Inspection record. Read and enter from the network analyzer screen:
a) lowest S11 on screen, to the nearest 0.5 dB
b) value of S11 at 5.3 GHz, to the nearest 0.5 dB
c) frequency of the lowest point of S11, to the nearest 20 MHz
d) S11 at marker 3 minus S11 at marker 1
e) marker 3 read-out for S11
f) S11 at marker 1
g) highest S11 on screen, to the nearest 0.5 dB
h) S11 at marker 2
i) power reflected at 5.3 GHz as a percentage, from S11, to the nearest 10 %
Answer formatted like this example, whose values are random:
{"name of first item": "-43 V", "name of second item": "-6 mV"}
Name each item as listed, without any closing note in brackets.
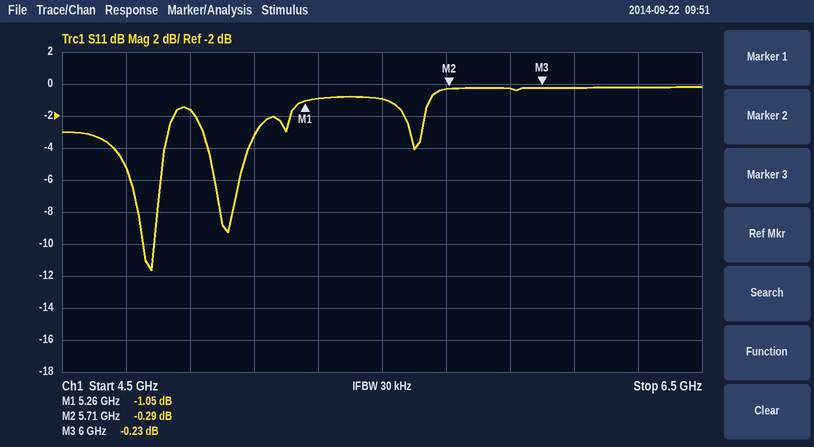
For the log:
{"lowest S11 on screen, to the nearest 0.5 dB": "-11.5 dB", "value of S11 at 5.3 GHz, to the nearest 0.5 dB": "-1.0 dB", "frequency of the lowest point of S11, to the nearest 20 MHz": "4.78 GHz", "S11 at marker 3 minus S11 at marker 1": "0.82 dB", "marker 3 read-out for S11": "-0.23 dB", "S11 at marker 1": "-1.05 dB", "highest S11 on screen, to the nearest 0.5 dB": "0.0 dB", "S11 at marker 2": "-0.29 dB", "power reflected at 5.3 GHz as a percentage, from S11, to the nearest 10 %": "80 %"}
